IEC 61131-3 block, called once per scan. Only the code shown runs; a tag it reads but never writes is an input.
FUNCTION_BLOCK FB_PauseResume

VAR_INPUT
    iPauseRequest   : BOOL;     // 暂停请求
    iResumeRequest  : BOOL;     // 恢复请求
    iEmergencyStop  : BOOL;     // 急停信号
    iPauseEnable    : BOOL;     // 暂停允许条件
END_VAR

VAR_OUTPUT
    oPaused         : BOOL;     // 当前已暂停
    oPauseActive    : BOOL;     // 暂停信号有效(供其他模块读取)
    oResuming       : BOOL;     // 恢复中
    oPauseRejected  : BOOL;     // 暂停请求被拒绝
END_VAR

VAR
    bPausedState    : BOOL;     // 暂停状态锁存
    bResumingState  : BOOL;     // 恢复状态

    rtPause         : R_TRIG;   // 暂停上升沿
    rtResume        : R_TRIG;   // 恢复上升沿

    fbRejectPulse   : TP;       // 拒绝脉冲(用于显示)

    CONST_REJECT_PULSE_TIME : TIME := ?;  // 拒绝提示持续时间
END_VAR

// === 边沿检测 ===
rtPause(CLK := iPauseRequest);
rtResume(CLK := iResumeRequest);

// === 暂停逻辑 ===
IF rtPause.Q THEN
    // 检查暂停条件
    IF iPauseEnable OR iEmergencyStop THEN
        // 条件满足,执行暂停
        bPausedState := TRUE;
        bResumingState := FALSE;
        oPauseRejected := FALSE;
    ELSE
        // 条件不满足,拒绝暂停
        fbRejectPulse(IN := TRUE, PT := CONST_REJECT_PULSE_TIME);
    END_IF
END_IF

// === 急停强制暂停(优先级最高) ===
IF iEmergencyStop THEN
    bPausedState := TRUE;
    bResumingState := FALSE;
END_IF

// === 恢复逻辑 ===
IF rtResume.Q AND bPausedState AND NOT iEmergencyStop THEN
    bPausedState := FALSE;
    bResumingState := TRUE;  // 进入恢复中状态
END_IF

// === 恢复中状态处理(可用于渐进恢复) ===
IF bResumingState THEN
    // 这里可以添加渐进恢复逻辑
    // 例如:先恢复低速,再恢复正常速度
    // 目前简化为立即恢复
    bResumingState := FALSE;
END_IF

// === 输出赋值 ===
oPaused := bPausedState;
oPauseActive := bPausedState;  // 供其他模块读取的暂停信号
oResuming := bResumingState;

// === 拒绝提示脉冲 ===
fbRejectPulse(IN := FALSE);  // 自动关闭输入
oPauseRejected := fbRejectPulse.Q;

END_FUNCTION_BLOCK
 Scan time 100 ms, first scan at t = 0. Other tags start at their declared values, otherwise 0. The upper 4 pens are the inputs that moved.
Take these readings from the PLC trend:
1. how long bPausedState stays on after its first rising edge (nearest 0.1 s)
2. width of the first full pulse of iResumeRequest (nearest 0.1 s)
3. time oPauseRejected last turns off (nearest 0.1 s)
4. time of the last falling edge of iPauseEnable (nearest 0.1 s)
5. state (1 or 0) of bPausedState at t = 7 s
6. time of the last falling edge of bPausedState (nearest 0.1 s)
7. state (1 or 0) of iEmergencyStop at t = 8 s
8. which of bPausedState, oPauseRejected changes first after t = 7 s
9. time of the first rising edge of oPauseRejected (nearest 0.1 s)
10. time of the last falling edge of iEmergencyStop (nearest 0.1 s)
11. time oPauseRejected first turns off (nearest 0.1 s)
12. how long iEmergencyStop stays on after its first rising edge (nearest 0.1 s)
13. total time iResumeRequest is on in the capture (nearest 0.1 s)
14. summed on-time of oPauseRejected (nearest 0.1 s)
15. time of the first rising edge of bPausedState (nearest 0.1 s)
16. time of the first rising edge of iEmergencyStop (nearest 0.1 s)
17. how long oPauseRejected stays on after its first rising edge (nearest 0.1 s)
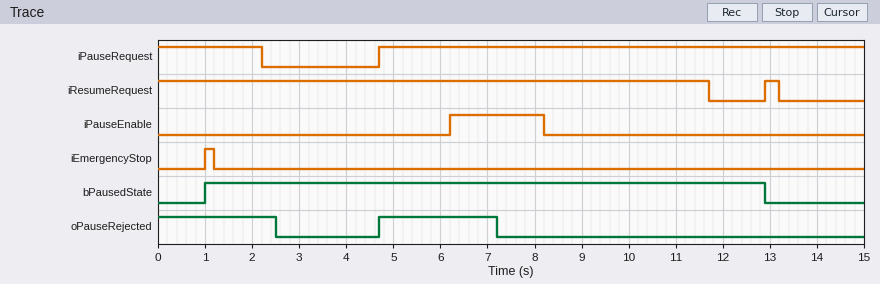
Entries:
11.9 s
0.3 s
7.2 s
8.2 s
1
12.9 s
0
oPauseRejected
4.7 s
1.2 s
2.5 s
0.2 s
12.0 s
5.0 s
1.0 s
1.0 s
2.5 s
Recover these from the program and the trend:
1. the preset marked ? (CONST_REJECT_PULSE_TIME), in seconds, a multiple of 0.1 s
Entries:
2.5 s
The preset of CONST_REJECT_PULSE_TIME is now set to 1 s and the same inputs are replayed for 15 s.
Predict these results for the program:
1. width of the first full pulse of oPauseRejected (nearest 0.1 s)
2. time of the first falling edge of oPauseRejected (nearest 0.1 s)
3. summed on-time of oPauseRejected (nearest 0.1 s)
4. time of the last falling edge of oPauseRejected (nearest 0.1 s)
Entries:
1.0 s
1.0 s
2.0 s
5.7 s
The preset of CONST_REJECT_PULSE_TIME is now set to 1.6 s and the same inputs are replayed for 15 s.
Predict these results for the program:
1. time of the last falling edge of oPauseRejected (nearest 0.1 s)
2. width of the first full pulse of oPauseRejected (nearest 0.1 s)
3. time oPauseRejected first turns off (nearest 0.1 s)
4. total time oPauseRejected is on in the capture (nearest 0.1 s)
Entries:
6.3 s
1.6 s
1.6 s
3.2 s
